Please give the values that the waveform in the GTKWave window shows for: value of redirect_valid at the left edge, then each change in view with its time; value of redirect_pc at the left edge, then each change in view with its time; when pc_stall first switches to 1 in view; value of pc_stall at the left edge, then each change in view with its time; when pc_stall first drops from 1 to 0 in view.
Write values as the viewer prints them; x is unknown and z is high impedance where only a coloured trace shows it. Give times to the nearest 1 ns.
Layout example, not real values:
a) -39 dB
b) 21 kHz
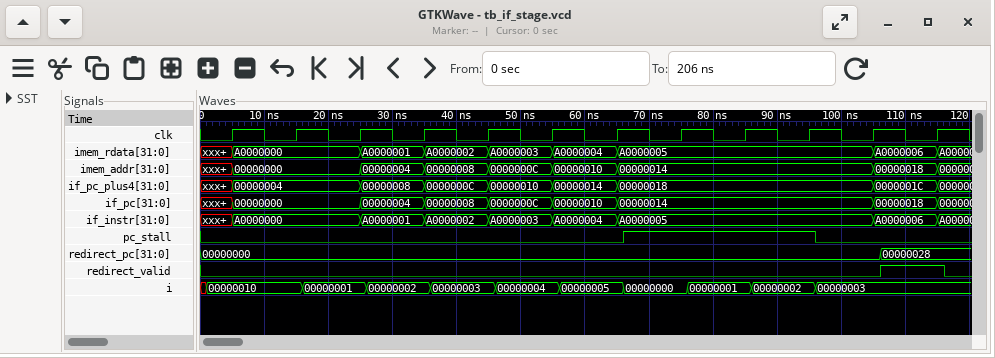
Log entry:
a) 0, 1 at 106 ns, 0 at 116 ns
b) 00000000, 00000028 at 106 ns
c) 66 ns
d) 0, 1 at 66 ns, 0 at 96 ns
e) 96 ns
